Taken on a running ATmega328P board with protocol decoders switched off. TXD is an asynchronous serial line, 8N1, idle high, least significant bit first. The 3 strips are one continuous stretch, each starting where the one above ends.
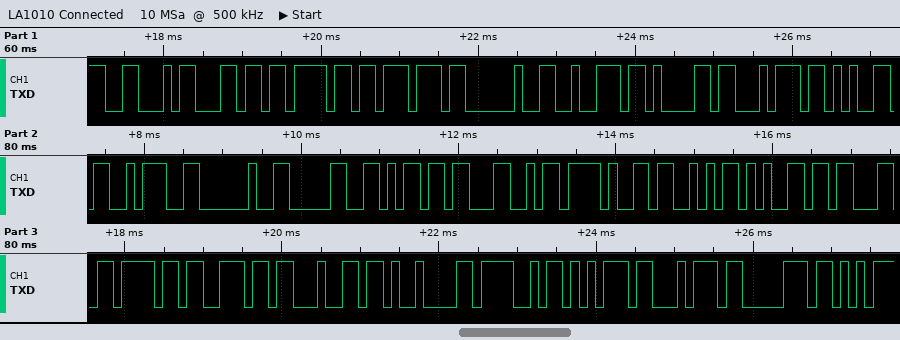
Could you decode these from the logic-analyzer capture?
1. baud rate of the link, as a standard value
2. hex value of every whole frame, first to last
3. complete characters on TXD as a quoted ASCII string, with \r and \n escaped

9600 baud
46 6C 6F 77 20 72 61 74 65 3A 20 30 6D 4C 2F 53 65 63 6F 6E 64 09 4F 75 74 70
"Flow rate: 0mL/Second\tOutp"
